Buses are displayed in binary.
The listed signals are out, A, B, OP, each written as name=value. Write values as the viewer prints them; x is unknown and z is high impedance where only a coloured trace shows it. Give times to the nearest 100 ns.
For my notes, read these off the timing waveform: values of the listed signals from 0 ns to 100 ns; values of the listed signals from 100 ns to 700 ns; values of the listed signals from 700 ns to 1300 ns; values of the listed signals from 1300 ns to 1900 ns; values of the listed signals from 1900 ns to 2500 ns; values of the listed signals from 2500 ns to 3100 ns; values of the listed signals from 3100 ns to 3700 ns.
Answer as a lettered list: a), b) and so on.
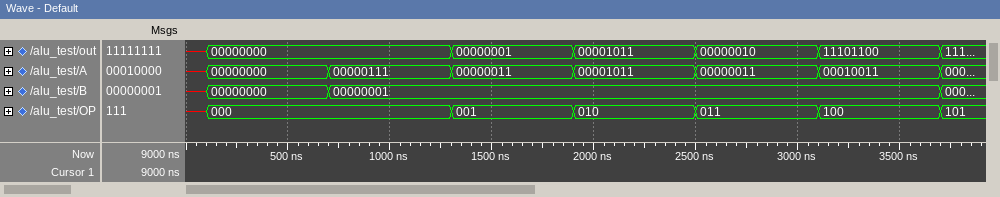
a) out=x, A=x, B=x, OP=x
b) out=00000000, A=00000000, B=00000000, OP=000
c) out=00000000, A=00000111, B=00000001, OP=000
d) out=00000001, A=00000011, B=00000001, OP=001
e) out=00001011, A=00001011, B=00000001, OP=010
f) out=00000010, A=00000011, B=00000001, OP=011
g) out=11101100, A=00010011, B=00000001, OP=100
